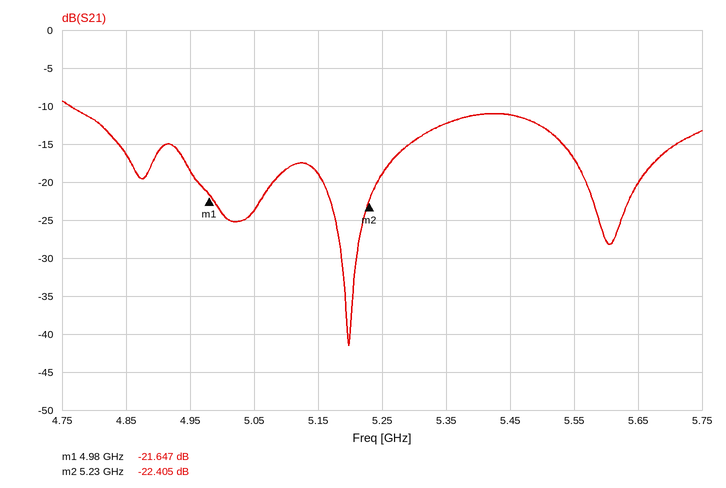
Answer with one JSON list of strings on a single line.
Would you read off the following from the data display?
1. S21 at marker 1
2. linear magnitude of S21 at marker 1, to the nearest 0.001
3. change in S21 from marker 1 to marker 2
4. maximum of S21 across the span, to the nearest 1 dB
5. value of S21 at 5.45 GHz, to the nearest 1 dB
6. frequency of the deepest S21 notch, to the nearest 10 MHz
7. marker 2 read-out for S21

["-21.647 dB", "0.083", "-0.758 dB", "-9 dB", "-11 dB", "5.20 GHz", "-22.405 dB"]
